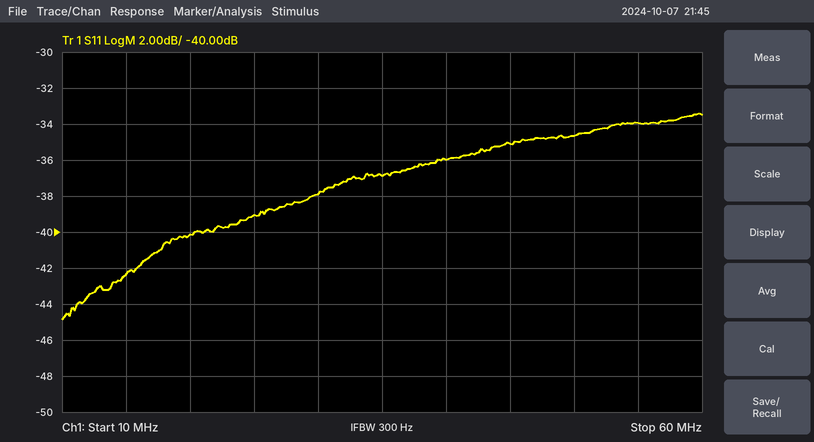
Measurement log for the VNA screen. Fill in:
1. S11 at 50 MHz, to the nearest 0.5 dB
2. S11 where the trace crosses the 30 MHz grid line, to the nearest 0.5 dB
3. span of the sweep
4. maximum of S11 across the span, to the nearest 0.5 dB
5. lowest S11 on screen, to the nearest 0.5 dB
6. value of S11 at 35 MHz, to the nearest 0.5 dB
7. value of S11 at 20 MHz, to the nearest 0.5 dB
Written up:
-34.5 dB
-38.0 dB
50 MHz
-33.5 dB
-45.0 dB
-37.0 dB
-40.0 dB
